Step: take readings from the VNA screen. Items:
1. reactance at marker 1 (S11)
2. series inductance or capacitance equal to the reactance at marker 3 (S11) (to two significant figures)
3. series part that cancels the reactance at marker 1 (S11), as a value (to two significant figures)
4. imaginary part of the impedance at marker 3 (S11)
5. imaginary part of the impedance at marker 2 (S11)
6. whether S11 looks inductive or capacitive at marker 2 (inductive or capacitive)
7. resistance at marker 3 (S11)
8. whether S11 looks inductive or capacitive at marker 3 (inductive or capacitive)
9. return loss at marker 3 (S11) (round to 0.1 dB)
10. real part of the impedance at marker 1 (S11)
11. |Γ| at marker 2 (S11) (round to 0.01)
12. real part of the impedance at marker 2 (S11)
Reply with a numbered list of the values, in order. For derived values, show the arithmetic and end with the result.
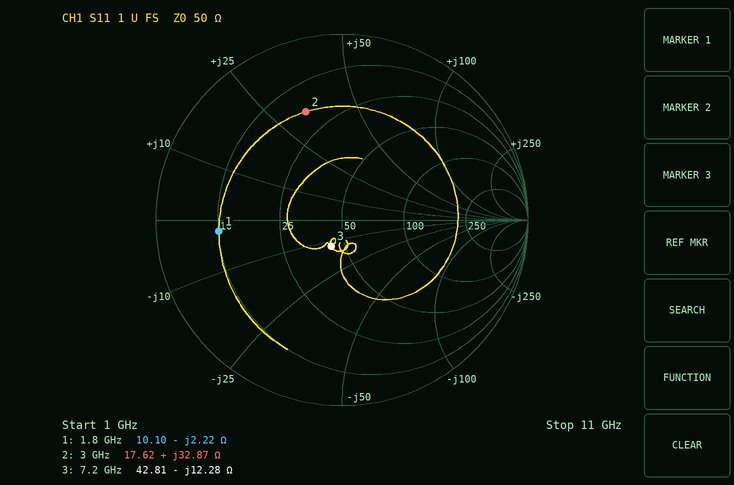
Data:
1. -2.22 Ω
2. C = 1/(2π × 7.2 GHz × 12.28 Ω) ≈ 1.8 pF
3. L = 2.22 Ω/(2π × 1.8 GHz) ≈ 196 pH, so 200 pH to two significant figures
4. -12.28 Ω
5. +32.87 Ω
6. inductive
7. 42.81 Ω
8. capacitive
9. 16.4 dB
10. 10.10 Ω
11. 0.61
12. 17.62 Ω
